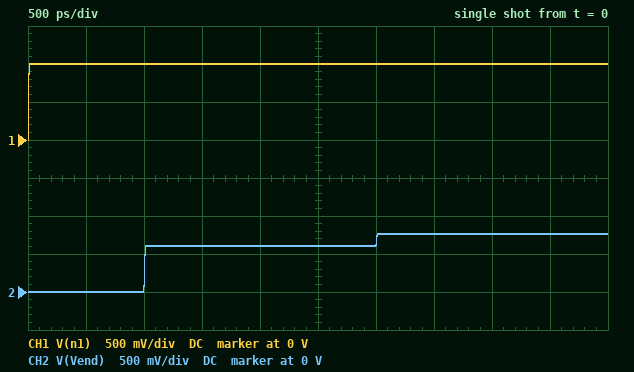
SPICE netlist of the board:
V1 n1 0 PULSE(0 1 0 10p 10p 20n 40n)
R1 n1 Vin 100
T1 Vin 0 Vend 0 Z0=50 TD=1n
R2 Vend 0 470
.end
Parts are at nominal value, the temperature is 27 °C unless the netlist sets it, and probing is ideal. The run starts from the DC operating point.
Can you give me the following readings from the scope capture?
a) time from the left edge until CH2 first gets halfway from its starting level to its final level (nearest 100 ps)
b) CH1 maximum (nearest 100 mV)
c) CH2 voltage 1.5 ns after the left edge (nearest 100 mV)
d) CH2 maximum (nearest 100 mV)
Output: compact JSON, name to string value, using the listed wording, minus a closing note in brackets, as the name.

{"time from the left edge until CH2 first gets halfway from its starting level to its final level": "1.0 ns", "CH1 maximum": "1.0 V", "CH2 voltage 1.5 ns after the left edge": "600 mV", "CH2 maximum": "800 mV"}
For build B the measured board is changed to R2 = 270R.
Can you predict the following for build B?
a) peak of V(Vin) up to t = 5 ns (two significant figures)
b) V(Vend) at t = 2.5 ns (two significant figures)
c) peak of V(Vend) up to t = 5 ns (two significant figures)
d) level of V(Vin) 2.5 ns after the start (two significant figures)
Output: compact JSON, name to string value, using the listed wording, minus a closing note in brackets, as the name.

{"peak of V(Vin) up to t = 5 ns": "710 mV", "V(Vend) at t = 2.5 ns": "560 mV", "peak of V(Vend) up to t = 5 ns": "690 mV", "level of V(Vin) 2.5 ns after the start": "640 mV"}
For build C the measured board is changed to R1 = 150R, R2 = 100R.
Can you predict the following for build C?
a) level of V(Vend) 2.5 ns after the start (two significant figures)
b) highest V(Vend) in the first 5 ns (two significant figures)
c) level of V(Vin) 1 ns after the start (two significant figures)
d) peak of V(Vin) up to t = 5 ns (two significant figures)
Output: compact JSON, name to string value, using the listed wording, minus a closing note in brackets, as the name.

{"level of V(Vend) 2.5 ns after the start": "330 mV", "highest V(Vend) in the first 5 ns": "390 mV", "level of V(Vin) 1 ns after the start": "250 mV", "peak of V(Vin) up to t = 5 ns": "400 mV"}
